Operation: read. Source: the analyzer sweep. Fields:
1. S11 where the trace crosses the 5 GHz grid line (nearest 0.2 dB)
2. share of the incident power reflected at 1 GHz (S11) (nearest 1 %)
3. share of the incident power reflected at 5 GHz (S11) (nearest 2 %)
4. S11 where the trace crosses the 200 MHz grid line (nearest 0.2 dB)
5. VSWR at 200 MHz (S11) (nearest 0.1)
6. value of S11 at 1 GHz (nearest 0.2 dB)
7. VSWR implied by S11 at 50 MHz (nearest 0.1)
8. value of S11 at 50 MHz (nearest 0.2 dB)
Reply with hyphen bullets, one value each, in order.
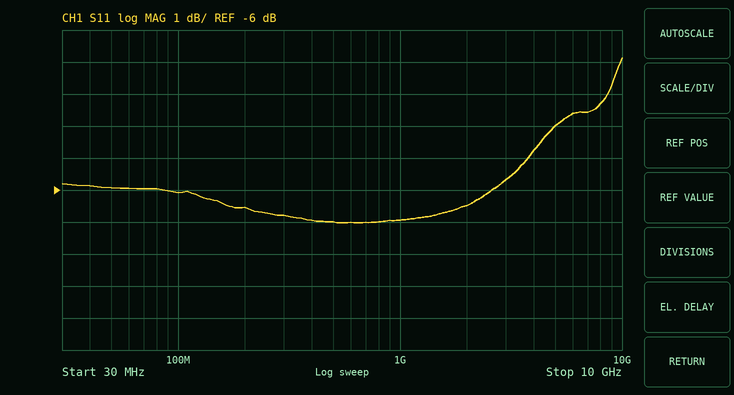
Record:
- -4.0 dB
- 20 %
- 40 %
- -6.6 dB
- 2.8
- -7.0 dB
- 3.0
- -6.0 dB
